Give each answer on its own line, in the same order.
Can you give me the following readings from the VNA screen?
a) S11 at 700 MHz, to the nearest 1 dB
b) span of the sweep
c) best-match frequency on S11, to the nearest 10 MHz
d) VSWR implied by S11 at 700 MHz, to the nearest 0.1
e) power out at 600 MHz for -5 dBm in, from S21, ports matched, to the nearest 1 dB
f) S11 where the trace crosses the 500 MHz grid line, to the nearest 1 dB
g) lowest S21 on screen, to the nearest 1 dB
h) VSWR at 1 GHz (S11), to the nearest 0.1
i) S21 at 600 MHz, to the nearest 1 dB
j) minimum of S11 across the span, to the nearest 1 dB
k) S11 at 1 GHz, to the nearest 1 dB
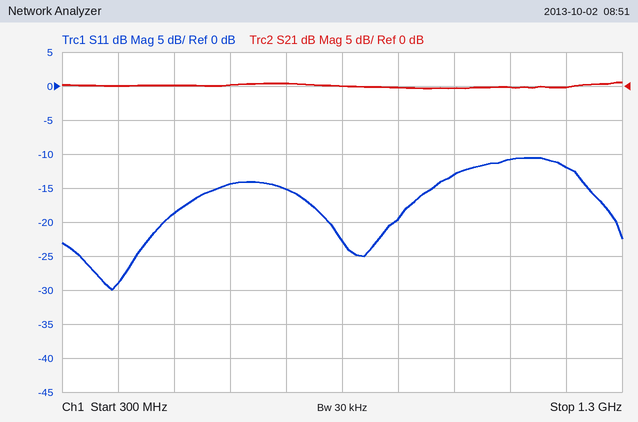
-15 dB
1 GHz
390 MHz
1.4
-5 dBm
-19 dB
0 dB
1.6
0 dB
-30 dB
-13 dB
